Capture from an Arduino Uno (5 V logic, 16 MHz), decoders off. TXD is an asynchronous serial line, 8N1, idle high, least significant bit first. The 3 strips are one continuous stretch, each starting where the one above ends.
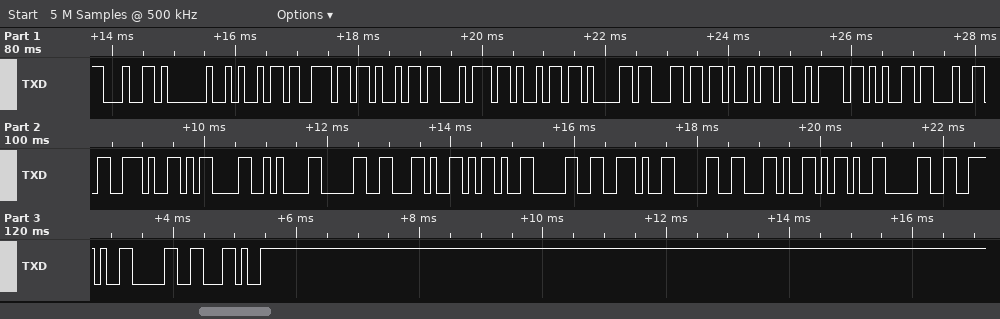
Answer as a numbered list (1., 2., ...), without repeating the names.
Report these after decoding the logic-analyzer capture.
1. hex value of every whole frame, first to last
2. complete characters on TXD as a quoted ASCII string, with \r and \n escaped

1. 64 20 69 6E 69 74 69 61 6C 69 7A 65 64 2E 0D 0A 30 2C 2D 30 2E 30 2C 2D 30 2E 30 2C
2. "d initialized.\r\n0,-0.0,-0.0,"
